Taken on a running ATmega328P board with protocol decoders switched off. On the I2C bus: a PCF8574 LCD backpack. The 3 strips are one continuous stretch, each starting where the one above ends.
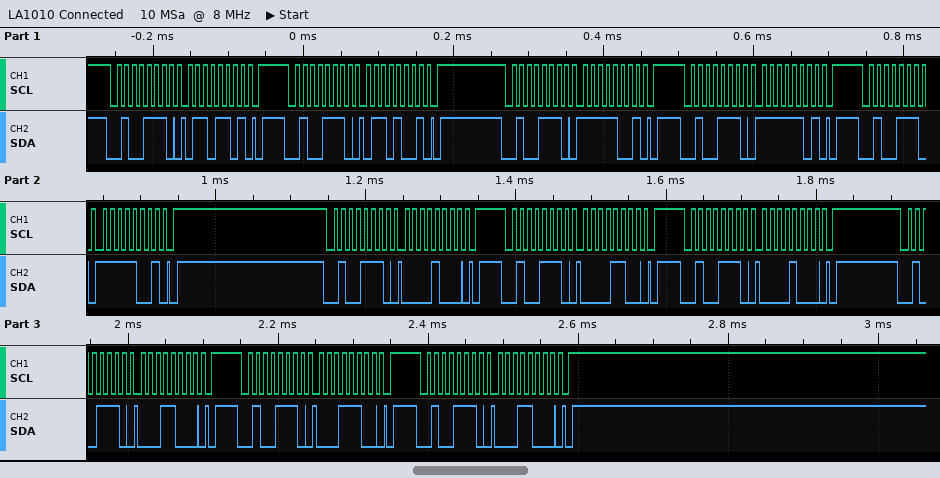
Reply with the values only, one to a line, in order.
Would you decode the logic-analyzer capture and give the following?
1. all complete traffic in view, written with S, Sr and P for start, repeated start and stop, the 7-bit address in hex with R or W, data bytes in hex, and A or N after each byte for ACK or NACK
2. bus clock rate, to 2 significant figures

S 27W A 6D A P S 27W A 69 A P S 27W A F9 A P S 27W A FD A P S 27W A F9 A P S 27W A 08 A P S 27W A 0C A P S 27W A 08 A P S 27W A 18 A P S 27W A 1C A P S 27W A 18 A P
100 kHz
